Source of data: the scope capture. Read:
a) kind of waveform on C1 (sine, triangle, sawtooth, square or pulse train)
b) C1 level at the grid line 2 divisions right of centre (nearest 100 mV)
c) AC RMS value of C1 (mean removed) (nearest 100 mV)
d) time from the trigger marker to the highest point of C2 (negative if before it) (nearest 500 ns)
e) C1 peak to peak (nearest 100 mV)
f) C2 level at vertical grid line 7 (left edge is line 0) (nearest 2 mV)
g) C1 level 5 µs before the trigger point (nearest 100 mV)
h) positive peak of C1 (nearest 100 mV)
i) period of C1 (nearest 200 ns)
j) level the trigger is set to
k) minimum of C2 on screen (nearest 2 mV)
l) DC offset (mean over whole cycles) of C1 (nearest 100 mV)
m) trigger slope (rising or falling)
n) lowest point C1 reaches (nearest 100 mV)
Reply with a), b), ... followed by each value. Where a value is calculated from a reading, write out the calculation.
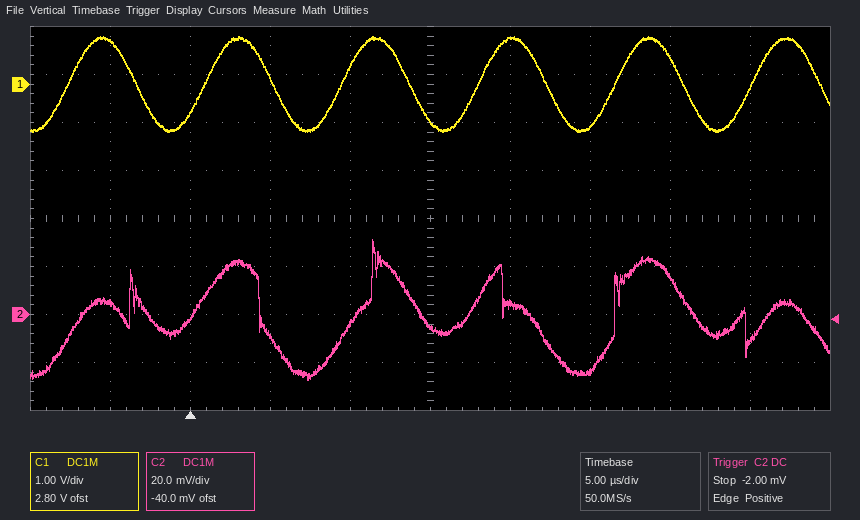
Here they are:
a) sine
b) -900 mV
c) 2.0 V / (2√2) ≈ 707 mV, so 700 mV to the nearest 100 mV
d) +11.5 µs
e) 1.0 V − (-1.0 V) = 2.0 V
f) -24 mV
g) 900 mV
h) 1.0 V
i) 8.6 µs
j) -2.00 mV
k) -28 mV
l) (1.0 V + (-1.0 V)) / 2 ≈ 0.0 V
m) rising
n) -1.0 V
